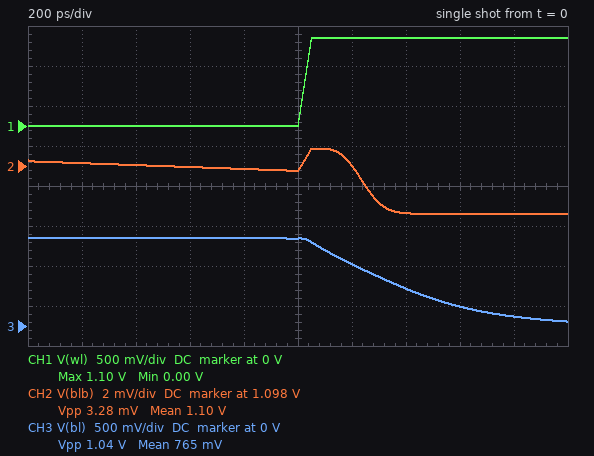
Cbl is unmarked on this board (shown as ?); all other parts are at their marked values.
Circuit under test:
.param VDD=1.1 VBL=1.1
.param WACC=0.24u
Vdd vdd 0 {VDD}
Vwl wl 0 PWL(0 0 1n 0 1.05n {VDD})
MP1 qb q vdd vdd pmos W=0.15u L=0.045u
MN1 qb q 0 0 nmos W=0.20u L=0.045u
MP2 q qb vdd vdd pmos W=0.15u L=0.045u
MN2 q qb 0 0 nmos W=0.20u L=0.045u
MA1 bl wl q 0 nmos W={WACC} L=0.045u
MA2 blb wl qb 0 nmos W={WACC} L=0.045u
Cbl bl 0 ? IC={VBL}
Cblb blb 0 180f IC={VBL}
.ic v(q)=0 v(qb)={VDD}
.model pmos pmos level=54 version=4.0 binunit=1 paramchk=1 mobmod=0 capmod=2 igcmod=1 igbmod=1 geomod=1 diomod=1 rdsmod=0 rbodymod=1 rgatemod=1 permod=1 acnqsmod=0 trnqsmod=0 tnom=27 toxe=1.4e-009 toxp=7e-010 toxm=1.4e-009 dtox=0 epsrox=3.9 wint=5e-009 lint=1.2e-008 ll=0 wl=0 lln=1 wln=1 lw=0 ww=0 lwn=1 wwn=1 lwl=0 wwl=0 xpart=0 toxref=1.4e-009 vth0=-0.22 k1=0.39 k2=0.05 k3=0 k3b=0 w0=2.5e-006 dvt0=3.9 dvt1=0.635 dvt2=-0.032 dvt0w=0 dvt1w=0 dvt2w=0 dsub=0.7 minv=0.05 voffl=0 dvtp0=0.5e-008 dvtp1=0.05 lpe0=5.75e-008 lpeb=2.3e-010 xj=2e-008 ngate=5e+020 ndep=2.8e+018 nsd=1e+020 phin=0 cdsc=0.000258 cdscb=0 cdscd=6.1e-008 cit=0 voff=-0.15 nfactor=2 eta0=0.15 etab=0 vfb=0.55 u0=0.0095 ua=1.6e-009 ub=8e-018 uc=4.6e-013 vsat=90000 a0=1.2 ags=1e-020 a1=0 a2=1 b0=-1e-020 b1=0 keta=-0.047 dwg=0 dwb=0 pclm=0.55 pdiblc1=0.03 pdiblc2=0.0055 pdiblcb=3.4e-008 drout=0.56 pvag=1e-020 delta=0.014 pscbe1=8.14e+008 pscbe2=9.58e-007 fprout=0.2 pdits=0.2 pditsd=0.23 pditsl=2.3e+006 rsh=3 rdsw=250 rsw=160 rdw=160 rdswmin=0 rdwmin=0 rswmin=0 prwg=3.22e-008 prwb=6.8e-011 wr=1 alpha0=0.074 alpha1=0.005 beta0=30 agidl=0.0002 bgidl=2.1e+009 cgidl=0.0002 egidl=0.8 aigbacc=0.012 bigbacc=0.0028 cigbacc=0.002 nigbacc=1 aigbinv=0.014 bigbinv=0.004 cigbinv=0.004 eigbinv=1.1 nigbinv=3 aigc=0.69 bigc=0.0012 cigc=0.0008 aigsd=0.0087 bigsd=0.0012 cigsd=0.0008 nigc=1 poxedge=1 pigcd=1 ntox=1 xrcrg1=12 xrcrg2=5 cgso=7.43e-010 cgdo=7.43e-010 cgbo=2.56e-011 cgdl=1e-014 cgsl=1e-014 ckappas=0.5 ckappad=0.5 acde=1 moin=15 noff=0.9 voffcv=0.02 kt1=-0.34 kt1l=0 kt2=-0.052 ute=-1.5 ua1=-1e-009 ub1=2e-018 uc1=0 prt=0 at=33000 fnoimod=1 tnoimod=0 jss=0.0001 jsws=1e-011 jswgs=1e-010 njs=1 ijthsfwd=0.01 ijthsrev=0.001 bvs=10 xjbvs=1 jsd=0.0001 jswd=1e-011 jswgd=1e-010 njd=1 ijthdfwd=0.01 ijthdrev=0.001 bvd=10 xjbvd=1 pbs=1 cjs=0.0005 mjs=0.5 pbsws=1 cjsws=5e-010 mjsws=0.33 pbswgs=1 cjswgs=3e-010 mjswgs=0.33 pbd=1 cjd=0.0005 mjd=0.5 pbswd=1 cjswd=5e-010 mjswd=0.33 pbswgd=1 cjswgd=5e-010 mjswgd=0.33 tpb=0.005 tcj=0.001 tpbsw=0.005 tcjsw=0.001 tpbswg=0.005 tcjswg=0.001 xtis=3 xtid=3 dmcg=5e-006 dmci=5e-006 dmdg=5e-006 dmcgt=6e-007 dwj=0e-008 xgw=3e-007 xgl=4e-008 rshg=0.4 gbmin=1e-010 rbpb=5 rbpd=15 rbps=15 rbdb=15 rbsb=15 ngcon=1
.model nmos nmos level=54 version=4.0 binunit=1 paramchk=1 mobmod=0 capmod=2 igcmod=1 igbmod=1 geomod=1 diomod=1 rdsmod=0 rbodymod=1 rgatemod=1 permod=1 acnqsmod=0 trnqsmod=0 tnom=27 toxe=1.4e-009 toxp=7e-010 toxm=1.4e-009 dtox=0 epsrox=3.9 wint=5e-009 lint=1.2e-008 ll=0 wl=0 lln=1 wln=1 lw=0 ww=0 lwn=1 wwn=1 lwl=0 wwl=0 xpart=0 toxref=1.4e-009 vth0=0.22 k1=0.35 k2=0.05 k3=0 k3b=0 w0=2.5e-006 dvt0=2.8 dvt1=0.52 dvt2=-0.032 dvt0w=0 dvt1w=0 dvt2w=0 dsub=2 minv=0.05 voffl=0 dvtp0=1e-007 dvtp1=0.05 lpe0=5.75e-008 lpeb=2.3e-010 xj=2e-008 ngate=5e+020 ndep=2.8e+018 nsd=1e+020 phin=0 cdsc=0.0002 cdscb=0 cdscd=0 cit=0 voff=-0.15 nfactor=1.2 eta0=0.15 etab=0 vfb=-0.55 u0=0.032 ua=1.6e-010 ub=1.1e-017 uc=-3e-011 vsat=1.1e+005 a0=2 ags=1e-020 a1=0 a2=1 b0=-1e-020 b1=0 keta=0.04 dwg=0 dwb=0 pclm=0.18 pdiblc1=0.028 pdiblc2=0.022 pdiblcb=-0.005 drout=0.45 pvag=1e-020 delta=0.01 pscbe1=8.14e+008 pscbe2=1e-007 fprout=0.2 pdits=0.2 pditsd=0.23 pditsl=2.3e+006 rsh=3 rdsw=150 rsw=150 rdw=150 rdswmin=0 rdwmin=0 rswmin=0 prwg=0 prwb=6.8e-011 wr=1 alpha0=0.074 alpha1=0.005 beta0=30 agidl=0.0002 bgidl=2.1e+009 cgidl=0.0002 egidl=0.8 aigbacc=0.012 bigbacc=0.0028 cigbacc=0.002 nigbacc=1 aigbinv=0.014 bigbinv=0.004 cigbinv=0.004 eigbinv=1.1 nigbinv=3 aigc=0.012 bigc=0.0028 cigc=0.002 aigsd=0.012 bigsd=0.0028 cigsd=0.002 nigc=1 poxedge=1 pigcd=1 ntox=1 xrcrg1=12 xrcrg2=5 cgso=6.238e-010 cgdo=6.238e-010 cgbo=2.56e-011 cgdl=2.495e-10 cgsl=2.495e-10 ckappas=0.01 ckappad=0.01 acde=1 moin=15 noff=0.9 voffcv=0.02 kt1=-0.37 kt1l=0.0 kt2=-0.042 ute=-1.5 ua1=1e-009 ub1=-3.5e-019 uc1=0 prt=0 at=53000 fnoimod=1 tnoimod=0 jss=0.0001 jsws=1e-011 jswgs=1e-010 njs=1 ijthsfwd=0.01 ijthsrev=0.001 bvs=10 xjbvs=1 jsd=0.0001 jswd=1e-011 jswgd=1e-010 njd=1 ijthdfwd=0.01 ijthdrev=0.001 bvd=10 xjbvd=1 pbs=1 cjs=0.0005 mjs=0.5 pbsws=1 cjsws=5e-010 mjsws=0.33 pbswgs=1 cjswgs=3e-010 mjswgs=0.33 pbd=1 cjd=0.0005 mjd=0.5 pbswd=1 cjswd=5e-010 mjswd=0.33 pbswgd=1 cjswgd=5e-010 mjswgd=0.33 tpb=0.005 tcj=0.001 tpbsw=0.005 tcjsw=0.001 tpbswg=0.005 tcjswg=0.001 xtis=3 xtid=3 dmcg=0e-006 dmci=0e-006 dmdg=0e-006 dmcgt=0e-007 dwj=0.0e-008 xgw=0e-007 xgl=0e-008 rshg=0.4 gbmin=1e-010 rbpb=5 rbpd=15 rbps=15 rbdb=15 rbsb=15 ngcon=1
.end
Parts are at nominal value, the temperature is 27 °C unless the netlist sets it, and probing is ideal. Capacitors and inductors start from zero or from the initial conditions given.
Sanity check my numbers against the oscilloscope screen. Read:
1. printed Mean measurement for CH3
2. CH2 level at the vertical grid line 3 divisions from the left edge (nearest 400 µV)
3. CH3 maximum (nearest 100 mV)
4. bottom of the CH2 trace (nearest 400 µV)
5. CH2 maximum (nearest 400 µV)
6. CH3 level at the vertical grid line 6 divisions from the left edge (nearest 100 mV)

765 mV
1.0980 V
1.1 V
1.0956 V
1.0988 V
800 mV
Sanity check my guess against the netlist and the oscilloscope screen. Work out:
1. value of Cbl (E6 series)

68 fF
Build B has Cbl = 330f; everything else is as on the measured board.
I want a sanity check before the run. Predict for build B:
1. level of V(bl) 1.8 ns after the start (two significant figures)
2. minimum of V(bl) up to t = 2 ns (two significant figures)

880 mV
840 mV
